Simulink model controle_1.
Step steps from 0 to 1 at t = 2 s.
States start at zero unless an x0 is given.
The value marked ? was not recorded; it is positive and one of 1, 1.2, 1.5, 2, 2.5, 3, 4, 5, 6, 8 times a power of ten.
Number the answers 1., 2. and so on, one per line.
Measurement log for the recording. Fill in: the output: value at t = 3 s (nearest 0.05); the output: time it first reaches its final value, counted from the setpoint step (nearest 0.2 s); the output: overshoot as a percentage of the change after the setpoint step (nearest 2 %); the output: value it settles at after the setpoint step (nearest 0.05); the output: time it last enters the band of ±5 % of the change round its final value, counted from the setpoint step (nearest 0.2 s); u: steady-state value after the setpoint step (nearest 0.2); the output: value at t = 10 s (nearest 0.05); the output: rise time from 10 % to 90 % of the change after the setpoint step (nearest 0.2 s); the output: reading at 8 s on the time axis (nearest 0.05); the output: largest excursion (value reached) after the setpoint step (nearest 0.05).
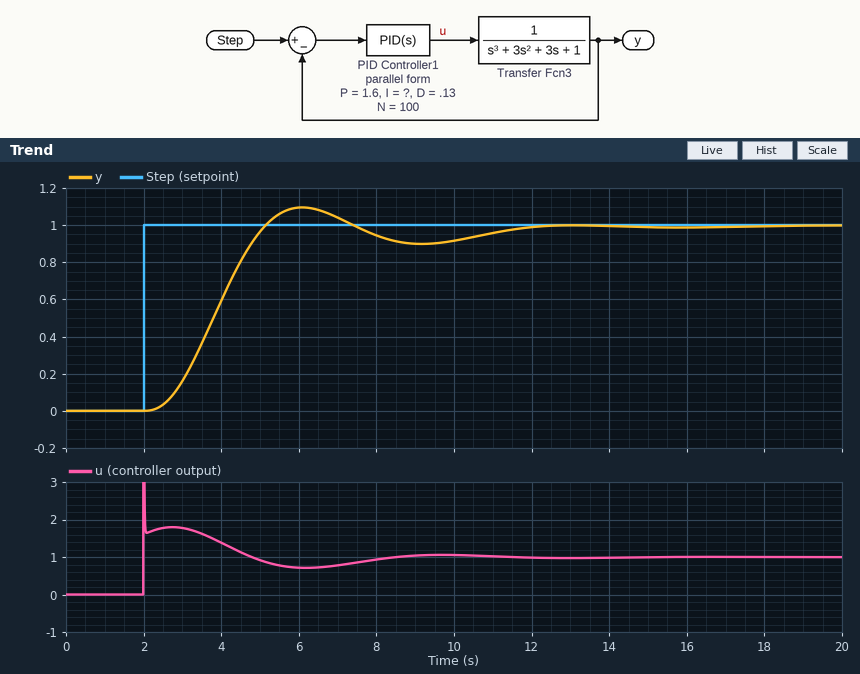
1. 0.15
2. 3.2 s
3. 10 %
4. 1.00
5. 8.8 s
6. 1.0
7. 0.90
8. 2.0 s
9. 0.95
10. 1.10
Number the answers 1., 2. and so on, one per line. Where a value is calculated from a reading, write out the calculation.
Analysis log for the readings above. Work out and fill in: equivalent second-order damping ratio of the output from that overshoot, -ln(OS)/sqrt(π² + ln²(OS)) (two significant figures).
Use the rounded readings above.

1. ln(0.1) = -2.303; 2.303 / sqrt(9.870 + 5.302) = 0.59
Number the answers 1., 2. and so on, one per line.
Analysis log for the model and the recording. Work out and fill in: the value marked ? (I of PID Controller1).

1. 0.5
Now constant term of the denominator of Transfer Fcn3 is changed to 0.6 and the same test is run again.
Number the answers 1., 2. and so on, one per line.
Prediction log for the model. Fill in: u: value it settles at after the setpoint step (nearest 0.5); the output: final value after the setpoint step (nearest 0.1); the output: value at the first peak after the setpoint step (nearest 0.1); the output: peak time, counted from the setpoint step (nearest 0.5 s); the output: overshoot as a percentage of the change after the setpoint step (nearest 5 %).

1. 0.5
2. 1.0
3. 1.2
4. 4.5 s
5. 25 %
